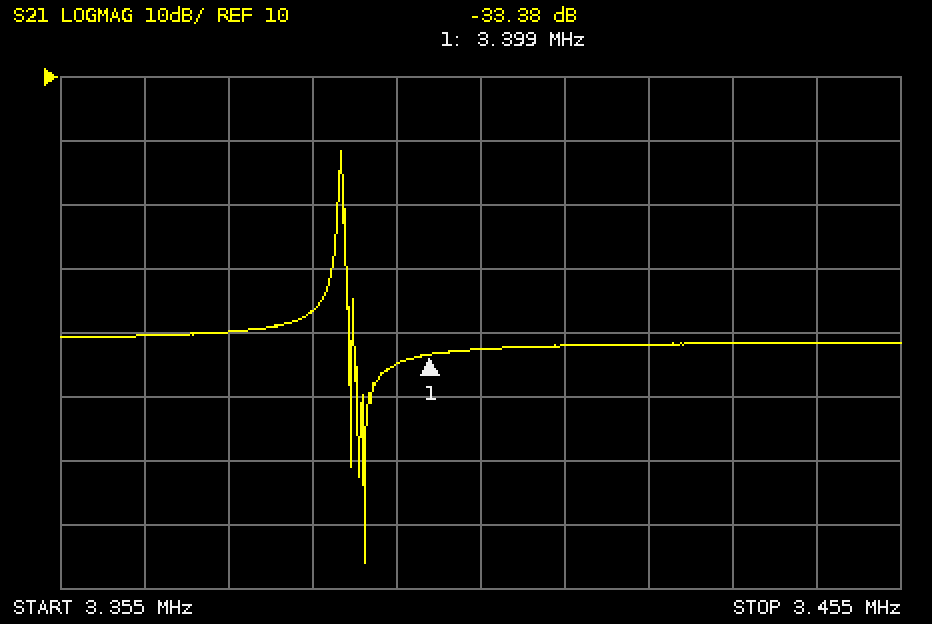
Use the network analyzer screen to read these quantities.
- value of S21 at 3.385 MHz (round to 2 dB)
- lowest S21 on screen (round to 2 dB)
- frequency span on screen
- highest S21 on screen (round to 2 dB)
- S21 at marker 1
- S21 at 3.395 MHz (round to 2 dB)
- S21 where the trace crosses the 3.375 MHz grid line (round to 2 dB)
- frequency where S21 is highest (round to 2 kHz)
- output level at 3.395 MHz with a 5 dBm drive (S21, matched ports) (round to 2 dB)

-26 dB
-66 dB
100 kHz
-2 dB
-33.38 dB
-34 dB
-30 dB
3.388 MHz
-30 dBm
